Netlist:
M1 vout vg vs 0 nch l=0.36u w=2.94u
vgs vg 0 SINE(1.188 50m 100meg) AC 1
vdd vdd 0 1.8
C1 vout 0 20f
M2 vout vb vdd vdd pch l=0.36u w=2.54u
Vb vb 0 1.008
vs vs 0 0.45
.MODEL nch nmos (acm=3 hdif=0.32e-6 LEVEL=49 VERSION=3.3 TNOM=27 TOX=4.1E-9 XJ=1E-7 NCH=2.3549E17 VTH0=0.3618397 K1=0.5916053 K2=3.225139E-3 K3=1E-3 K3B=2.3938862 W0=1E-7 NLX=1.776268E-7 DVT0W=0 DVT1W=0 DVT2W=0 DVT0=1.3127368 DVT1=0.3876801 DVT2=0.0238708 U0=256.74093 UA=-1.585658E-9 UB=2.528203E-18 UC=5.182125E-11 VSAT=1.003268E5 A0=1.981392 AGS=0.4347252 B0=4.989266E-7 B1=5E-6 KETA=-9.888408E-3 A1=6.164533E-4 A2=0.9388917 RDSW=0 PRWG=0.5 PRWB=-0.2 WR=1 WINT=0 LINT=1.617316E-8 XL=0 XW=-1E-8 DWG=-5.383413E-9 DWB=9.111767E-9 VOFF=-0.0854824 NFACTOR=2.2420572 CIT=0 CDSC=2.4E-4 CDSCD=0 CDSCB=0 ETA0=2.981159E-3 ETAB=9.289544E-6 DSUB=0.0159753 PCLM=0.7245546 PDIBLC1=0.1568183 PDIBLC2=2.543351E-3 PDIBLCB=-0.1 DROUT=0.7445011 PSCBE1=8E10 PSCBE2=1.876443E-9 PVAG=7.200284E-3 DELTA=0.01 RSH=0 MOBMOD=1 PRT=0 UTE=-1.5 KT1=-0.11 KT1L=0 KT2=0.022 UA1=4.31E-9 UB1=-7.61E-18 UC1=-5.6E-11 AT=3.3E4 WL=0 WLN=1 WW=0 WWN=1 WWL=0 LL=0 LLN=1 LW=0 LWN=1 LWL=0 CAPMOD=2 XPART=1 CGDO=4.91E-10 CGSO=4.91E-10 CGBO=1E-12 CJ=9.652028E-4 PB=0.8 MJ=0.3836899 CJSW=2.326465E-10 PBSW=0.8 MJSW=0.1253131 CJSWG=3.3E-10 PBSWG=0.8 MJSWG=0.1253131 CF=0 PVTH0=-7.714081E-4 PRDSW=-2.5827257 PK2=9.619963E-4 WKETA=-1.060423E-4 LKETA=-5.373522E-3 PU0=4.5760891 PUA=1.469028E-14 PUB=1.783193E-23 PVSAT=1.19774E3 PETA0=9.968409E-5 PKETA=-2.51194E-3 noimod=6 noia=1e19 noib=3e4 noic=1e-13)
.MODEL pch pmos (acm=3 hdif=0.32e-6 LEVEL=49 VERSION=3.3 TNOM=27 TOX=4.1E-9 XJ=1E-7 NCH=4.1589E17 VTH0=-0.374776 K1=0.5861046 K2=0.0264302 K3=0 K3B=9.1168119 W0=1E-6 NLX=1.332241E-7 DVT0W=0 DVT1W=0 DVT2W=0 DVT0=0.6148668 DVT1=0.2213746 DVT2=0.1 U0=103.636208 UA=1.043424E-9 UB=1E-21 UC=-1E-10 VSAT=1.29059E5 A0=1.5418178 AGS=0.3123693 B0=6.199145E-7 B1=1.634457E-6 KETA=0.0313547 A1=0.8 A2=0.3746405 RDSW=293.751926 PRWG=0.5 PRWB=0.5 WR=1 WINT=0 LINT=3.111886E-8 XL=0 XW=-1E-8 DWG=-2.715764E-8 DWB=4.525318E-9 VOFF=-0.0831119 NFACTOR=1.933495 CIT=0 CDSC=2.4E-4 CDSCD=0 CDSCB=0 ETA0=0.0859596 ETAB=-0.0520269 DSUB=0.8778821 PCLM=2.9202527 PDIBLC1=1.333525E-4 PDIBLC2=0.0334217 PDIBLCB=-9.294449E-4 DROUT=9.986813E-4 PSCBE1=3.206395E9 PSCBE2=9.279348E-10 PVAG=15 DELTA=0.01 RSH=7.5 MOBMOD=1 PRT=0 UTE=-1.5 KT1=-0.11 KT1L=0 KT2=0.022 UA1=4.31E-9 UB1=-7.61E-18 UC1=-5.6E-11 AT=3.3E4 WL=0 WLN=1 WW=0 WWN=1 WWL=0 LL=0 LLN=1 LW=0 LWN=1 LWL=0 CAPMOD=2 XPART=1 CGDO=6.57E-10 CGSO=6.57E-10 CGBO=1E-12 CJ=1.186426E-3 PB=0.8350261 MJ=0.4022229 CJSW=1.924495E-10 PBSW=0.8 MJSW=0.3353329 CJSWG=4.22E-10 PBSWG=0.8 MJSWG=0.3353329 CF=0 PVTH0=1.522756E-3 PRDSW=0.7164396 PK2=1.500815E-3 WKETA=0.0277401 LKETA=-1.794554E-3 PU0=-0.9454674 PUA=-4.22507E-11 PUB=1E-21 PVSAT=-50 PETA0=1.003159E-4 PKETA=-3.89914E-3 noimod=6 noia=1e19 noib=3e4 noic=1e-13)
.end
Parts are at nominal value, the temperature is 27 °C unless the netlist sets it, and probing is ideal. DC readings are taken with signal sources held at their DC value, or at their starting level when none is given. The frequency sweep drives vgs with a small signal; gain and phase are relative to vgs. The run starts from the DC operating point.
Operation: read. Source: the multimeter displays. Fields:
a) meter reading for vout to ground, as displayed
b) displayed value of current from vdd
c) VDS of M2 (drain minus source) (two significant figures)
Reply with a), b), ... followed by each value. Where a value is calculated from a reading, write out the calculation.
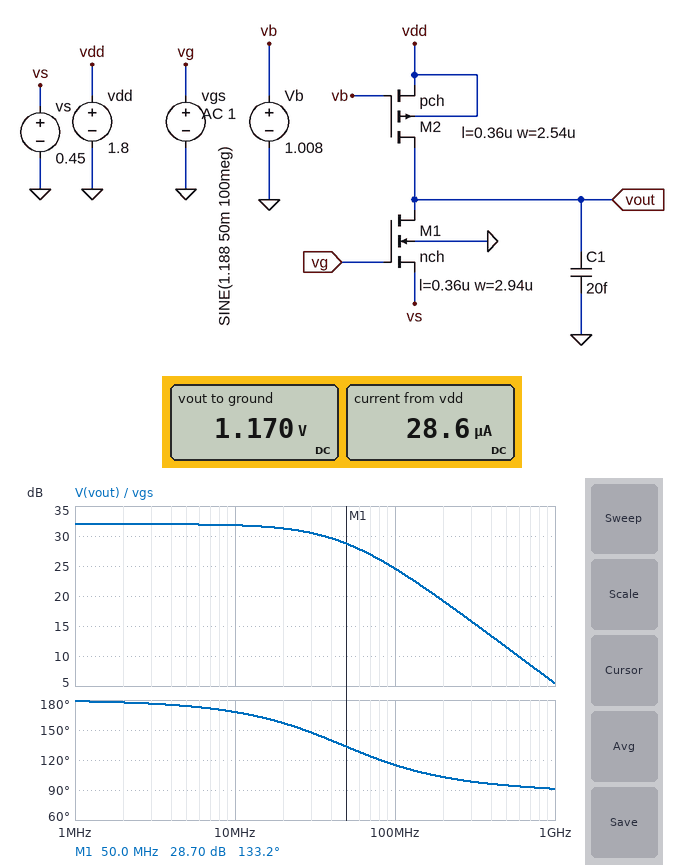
a) 1.170 V
b) 28.6 µA
c) 1.17 V - 1.8 V = -630 mV
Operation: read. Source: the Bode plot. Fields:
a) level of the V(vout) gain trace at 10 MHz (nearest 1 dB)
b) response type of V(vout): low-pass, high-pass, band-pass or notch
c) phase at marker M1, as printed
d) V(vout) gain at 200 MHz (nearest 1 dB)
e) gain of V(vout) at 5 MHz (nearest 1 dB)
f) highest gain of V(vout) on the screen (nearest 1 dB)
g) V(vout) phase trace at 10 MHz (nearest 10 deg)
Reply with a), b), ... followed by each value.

a) 32 dB
b) low-pass
c) 133.2 deg
d) 19 dB
e) 32 dB
f) 32 dB
g) 170 deg
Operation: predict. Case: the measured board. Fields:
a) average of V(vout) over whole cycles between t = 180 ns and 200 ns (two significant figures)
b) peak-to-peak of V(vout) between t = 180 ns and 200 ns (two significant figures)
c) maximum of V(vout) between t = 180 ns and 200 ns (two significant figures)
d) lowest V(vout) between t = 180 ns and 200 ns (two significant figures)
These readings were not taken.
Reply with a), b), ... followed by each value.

a) 1.1 V
b) 1.1 V
c) 1.7 V
d) 540 mV
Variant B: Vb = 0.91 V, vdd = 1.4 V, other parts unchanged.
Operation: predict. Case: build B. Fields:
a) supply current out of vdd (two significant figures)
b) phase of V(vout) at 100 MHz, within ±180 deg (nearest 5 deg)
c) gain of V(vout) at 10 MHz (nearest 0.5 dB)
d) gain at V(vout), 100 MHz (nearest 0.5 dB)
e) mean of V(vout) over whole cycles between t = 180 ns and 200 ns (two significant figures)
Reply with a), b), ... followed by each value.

a) 1.1 µA
b) 155 deg
c) -31.5 dB
d) -31.0 dB
e) 450 mV
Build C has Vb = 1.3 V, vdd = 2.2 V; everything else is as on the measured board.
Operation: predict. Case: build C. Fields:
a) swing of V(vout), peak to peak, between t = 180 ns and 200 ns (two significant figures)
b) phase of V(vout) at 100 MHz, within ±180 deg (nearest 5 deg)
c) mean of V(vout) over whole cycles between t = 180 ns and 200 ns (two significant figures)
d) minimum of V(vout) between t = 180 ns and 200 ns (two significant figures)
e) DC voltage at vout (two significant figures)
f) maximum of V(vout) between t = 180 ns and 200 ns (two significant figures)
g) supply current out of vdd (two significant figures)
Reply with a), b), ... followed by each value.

a) 560 mV
b) 170 deg
c) 1.9 V
d) 1.6 V
e) 2.0 V
f) 2.1 V
g) 32 µA
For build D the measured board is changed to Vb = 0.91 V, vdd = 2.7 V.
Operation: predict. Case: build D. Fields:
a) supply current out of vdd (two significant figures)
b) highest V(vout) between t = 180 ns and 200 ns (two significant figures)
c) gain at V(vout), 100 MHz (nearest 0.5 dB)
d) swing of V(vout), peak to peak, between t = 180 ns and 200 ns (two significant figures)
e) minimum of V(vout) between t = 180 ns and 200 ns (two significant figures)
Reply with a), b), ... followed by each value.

a) 35 µA
b) 2.7 V
c) -3.0 dB
d) 70 mV
e) 2.6 V
